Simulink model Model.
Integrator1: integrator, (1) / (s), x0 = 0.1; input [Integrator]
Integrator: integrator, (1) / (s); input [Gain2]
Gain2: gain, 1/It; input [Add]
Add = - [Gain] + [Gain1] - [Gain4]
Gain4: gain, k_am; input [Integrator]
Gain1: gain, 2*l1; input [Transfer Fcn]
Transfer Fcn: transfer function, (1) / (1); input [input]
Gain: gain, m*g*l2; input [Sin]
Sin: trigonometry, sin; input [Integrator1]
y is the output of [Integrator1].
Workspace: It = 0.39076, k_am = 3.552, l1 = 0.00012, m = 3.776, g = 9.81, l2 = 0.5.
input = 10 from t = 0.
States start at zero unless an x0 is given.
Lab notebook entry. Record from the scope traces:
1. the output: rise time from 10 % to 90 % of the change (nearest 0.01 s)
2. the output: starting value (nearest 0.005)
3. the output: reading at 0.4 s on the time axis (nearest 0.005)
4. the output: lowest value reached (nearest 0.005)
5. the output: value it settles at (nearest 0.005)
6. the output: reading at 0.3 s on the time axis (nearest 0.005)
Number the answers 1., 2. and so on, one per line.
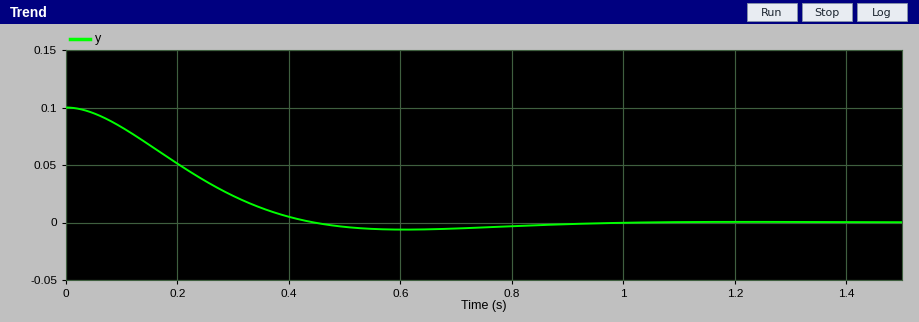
1. 0.29 s
2. 0.100
3. 0.005
4. -0.005
5. 0.000
6. 0.025
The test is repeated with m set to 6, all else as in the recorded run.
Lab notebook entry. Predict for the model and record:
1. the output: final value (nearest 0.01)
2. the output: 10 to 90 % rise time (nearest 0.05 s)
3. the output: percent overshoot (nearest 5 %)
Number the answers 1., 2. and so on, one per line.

1. 0.00
2. 0.20 s
3. 15 %
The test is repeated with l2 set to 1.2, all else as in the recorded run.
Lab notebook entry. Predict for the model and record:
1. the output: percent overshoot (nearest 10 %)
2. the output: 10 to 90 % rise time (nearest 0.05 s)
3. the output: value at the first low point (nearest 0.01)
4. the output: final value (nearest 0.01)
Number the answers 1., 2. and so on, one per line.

1. 20 %
2. 0.15 s
3. -0.02
4. 0.00
